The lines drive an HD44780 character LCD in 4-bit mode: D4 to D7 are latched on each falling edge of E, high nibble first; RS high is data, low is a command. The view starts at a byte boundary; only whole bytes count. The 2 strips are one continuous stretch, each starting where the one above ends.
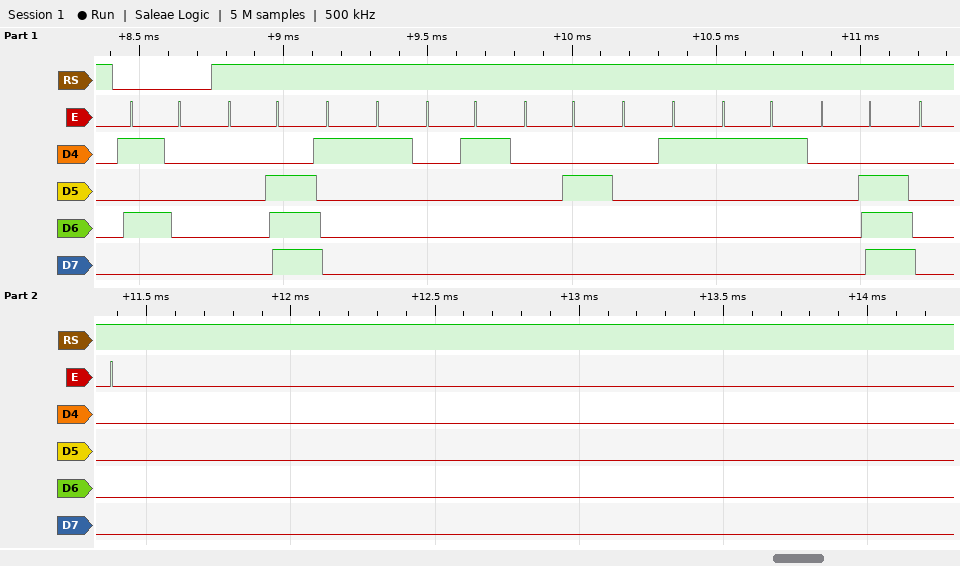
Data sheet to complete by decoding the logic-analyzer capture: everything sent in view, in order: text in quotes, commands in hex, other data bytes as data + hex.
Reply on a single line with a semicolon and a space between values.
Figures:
0x50 data 0E 11 01 02 01 11 0E 00
